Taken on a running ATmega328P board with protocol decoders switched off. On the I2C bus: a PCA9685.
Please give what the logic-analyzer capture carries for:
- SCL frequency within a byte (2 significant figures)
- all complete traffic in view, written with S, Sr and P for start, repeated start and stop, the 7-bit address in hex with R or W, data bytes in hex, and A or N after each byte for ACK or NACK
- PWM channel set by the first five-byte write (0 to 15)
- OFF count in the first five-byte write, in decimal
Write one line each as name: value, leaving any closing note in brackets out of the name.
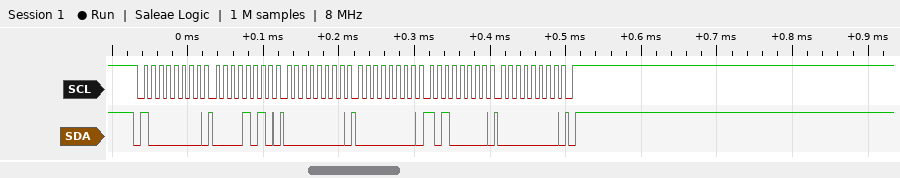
SCL frequency within a byte: 100 kHz
all complete traffic in view, written with S, Sr and P for start, repeated start and stop, the 7-bit address in hex with R or W, data bytes in hex, and A or N after each byte for ACK or NACK: S 40W A 0A A 00 A 00 A A0 A 00 A P
PWM channel set by the first five-byte write: 1
OFF count in the first five-byte write, in decimal: 160
